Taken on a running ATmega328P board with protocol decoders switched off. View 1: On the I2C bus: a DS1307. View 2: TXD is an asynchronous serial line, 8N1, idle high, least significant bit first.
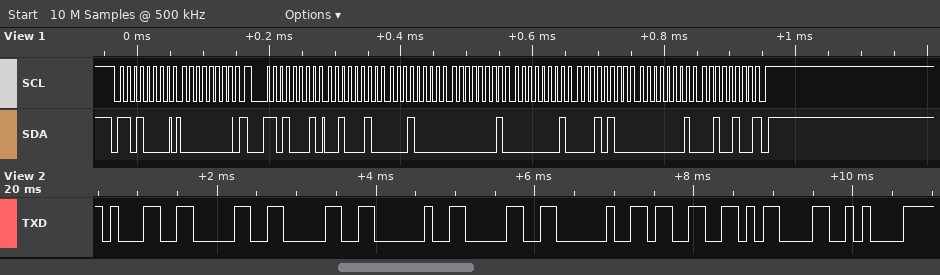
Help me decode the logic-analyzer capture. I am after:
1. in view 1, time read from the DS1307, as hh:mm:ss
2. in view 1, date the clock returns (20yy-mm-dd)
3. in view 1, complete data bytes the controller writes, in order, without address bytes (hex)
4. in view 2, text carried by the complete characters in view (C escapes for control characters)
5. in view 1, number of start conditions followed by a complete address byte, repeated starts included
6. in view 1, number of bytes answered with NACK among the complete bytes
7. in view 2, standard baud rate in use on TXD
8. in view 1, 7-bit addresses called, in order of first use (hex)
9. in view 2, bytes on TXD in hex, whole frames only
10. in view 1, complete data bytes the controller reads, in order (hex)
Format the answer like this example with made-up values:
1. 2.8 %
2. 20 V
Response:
1. 01:10:22
2. 2024-01-14
3. 00
4. "100 0 3\r\n"
5. 2
6. 1
7. 9600 baud
8. 0x68
9. 0x31 0x30 0x30 0x20 0x30 0x20 0x33 0x0D 0x0A
10. 22 10 01 01 14 01 24
